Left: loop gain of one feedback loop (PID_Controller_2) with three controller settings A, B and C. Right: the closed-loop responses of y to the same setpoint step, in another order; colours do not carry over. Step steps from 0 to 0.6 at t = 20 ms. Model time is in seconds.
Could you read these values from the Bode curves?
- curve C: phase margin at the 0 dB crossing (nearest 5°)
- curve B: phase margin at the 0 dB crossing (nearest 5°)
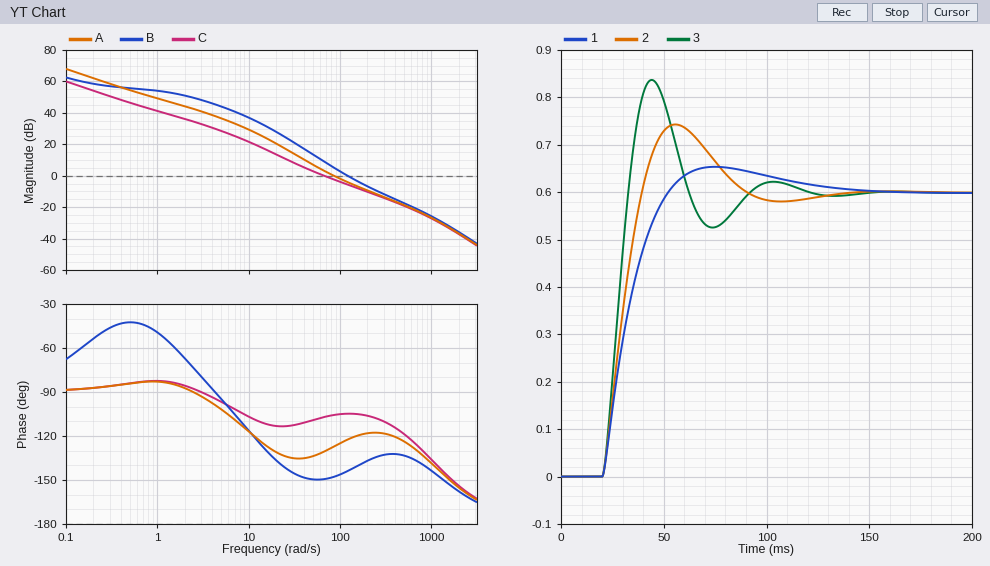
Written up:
75°
35°
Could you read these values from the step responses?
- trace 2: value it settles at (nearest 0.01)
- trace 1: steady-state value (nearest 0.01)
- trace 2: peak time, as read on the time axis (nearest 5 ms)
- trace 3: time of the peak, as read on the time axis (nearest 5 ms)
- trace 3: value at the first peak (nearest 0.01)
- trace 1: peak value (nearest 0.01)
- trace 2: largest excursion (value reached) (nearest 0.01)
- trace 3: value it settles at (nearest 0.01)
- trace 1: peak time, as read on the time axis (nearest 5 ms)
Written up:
0.60
0.60
55 ms
45 ms
0.84
0.65
0.74
0.60
75 ms
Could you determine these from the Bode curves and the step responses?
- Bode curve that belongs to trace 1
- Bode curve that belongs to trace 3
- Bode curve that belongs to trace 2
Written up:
C
B
A
